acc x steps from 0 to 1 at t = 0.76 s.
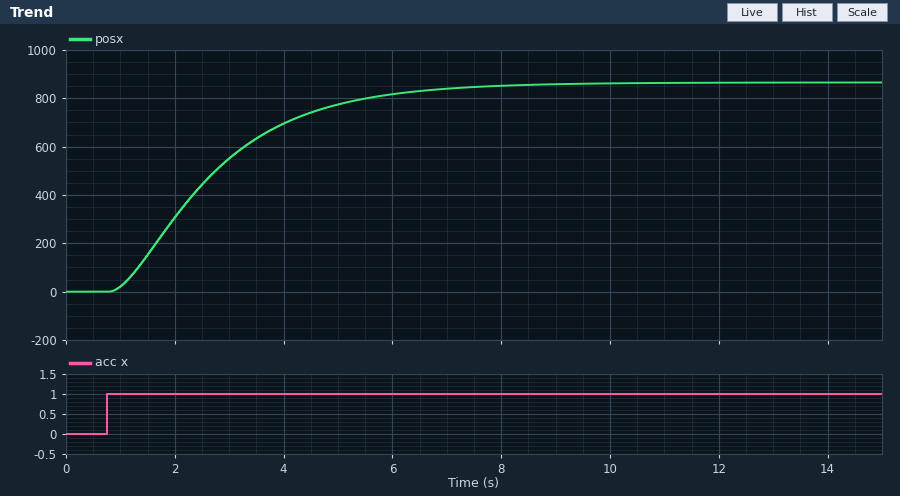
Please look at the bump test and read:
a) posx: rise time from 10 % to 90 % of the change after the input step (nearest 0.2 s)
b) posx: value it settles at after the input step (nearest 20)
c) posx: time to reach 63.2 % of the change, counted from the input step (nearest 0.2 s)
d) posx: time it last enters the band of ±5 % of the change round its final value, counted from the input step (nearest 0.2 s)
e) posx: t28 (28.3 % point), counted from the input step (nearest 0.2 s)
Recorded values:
3.8 s
860
2.2 s
5.4 s
1.0 s
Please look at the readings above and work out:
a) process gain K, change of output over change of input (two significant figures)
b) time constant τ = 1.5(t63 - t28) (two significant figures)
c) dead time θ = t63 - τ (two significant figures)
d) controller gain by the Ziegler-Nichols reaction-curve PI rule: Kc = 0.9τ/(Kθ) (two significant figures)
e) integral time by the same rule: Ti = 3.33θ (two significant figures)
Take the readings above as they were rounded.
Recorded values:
860
1.8 s
0.40 s
0.0047
1.3 s
